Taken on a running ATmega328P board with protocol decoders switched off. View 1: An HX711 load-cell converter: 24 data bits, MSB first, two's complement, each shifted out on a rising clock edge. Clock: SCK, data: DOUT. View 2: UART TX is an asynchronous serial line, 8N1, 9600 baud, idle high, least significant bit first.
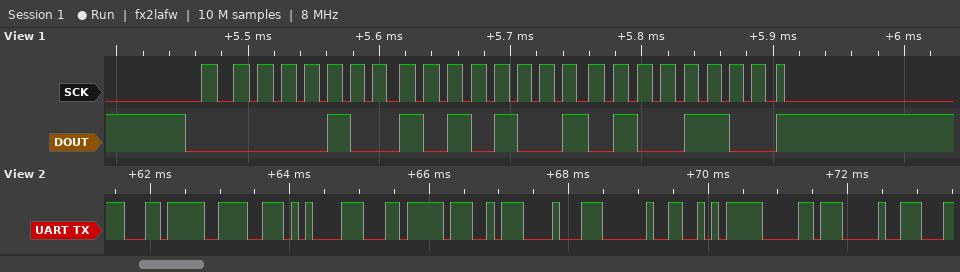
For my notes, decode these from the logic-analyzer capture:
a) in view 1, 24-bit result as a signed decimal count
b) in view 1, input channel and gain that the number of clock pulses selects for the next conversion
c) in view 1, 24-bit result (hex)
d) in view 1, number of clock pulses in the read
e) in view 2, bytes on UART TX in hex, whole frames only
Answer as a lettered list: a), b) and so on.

a) 305484
b) channel A, gain 128
c) 0x04A94C
d) 25
e) 0xEC 0x9E 0x85 0xEC 0xA7 0x88 0x20 0xEA 0xB0 0x90
